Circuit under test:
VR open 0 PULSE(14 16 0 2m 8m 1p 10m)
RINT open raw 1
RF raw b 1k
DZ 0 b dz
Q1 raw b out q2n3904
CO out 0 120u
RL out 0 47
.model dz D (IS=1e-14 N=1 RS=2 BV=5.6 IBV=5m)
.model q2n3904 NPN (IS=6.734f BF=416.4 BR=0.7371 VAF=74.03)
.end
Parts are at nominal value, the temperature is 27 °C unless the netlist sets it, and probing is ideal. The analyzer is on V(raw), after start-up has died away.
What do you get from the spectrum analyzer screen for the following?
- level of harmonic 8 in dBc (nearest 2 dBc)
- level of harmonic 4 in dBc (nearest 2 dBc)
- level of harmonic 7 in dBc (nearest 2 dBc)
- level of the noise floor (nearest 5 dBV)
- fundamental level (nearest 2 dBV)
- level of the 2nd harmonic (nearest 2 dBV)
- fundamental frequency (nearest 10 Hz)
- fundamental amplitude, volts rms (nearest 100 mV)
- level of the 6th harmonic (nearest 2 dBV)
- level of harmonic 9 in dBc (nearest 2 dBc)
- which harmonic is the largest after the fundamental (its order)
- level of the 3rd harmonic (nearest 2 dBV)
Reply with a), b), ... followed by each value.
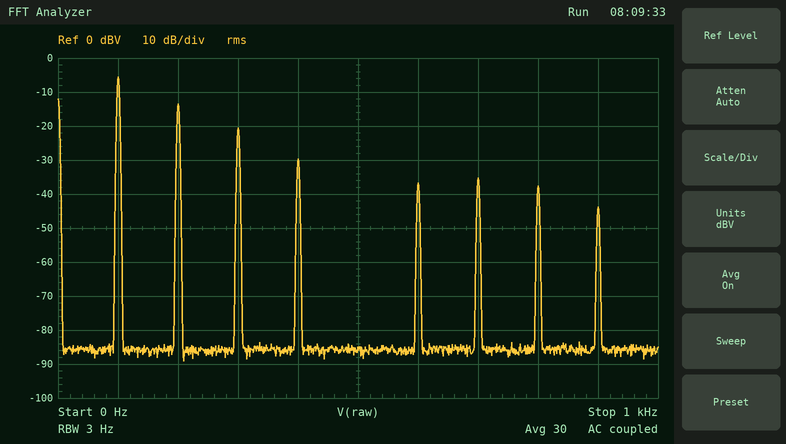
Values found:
a) -32 dBc
b) -24 dBc
c) -30 dBc
d) -85 dBV
e) -6 dBV
f) -14 dBV
g) 100 Hz
h) 500 mV
i) -36 dBV
j) -38 dBc
k) 2
l) -20 dBV
